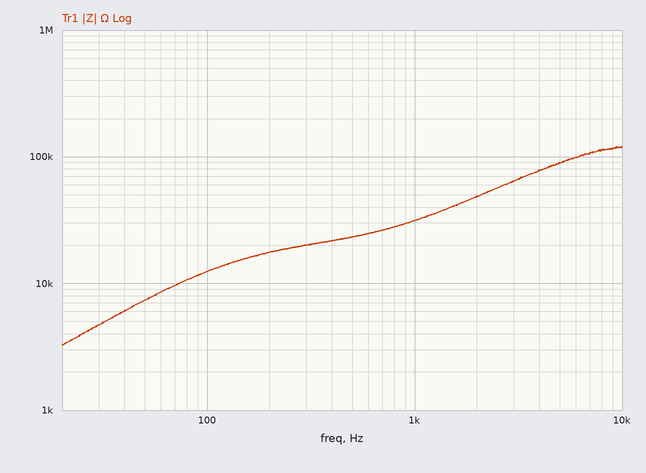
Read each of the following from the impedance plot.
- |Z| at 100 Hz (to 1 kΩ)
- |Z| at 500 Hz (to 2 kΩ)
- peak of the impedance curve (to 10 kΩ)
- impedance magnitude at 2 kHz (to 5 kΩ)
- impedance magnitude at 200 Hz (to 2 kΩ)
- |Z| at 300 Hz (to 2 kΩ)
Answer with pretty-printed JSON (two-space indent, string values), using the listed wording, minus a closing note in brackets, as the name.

{
  "|Z| at 100 Hz": "12 kΩ",
  "|Z| at 500 Hz": "24 kΩ",
  "peak of the impedance curve": "120 kΩ",
  "impedance magnitude at 2 kHz": "50 kΩ",
  "impedance magnitude at 200 Hz": "18 kΩ",
  "|Z| at 300 Hz": "20 kΩ"
}
